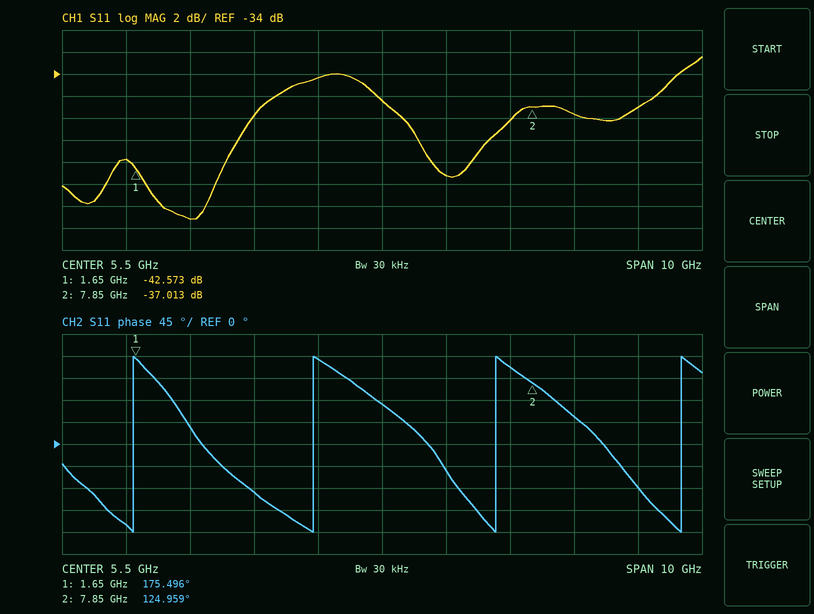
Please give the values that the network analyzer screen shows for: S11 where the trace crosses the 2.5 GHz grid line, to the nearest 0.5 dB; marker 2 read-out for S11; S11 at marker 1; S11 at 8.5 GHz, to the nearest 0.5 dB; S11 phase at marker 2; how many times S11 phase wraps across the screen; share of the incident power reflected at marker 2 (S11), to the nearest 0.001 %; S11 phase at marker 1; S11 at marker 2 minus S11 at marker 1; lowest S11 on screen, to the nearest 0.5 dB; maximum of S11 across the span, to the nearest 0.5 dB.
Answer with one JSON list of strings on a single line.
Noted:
["-47.0 dB", "-37.013 dB", "-42.573 dB", "-37.5 dB", "124.959°", "4", "0.020 %", "175.496°", "5.560 dB", "-47.0 dB", "-32.5 dB"]
